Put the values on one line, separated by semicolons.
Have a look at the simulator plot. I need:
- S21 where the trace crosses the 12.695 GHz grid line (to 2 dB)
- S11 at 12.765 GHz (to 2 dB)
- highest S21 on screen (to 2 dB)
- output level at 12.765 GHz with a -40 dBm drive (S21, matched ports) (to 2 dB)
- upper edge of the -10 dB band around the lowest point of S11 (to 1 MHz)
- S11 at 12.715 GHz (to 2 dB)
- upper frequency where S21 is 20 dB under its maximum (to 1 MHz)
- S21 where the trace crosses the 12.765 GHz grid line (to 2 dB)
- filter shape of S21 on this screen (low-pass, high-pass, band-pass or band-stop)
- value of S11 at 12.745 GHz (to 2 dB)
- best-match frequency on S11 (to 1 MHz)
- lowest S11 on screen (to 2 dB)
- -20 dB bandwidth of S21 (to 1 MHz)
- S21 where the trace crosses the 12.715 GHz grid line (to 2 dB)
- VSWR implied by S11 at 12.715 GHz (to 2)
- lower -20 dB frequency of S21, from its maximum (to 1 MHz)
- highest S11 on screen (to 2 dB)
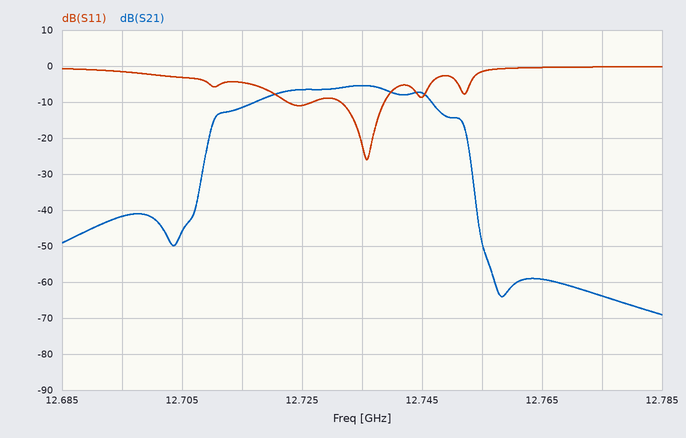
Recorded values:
-42 dB; 0 dB; -6 dB; -100 dBm; 12.739 GHz; -4 dB; 12.753 GHz; -60 dB; band-pass; -8 dB; 12.736 GHz; -26 dB; 44 MHz; -12 dB; 4; 12.709 GHz; 0 dB
